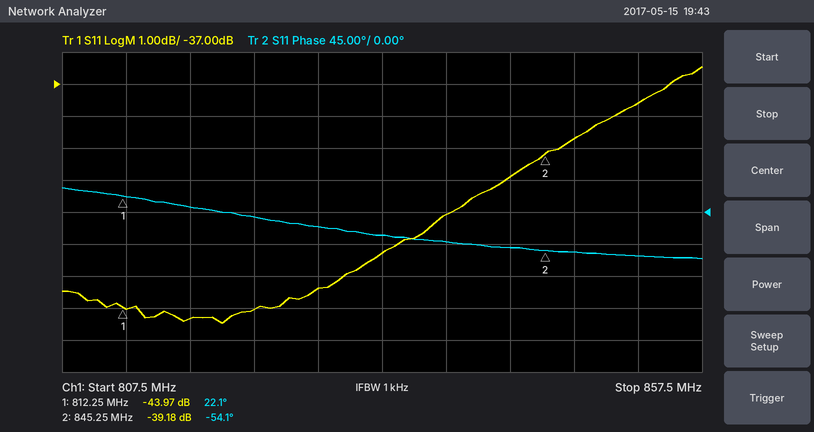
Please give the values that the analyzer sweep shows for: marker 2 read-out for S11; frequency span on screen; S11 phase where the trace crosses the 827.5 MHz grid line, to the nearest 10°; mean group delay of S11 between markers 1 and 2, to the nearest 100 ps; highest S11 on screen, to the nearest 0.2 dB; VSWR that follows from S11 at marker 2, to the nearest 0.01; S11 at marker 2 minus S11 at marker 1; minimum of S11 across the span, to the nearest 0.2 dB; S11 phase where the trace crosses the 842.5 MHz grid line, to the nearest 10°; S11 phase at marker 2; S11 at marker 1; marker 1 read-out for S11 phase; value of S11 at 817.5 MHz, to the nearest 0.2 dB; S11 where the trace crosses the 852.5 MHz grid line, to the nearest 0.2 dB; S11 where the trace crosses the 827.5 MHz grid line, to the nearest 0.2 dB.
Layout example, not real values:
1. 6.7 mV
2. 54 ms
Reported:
1. -39.18 dB
2. 50 MHz
3. -20°
4. 6.4 ns
5. -36.4 dB
6. 1.02
7. 4.79 dB
8. -44.4 dB
9. -50°
10. -54.1°
11. -43.97 dB
12. 22.1°
13. -44.4 dB
14. -37.6 dB
15. -43.4 dB
